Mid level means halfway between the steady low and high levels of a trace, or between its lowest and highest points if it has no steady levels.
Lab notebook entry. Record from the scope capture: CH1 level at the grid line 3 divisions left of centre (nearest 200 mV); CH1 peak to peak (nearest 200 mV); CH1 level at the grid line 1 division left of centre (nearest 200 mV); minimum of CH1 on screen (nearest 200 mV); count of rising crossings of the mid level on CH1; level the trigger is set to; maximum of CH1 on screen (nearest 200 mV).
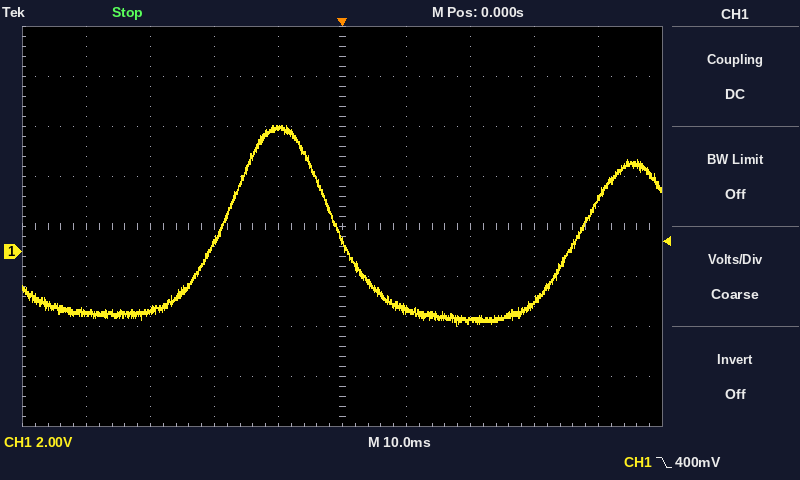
-2.4 V
8.0 V
5.0 V
-3.0 V
2
400 mV
5.0 V
